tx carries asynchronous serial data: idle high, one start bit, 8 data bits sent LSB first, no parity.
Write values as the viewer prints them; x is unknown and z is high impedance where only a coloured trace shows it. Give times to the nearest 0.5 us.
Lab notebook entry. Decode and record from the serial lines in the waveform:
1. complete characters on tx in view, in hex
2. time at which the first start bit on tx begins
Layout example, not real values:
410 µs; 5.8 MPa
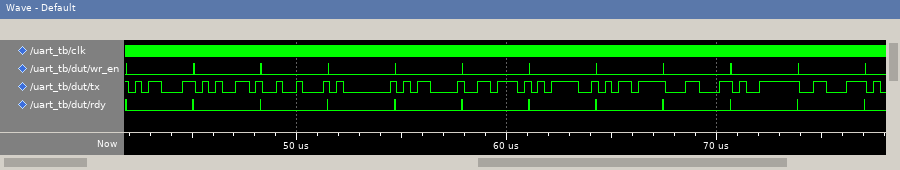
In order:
8D, 65, 12, 01, 0D, 76, 3D, ED, 8C, F9, C6; 42 us
